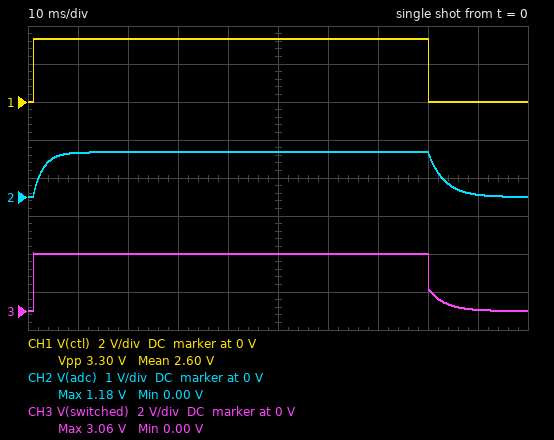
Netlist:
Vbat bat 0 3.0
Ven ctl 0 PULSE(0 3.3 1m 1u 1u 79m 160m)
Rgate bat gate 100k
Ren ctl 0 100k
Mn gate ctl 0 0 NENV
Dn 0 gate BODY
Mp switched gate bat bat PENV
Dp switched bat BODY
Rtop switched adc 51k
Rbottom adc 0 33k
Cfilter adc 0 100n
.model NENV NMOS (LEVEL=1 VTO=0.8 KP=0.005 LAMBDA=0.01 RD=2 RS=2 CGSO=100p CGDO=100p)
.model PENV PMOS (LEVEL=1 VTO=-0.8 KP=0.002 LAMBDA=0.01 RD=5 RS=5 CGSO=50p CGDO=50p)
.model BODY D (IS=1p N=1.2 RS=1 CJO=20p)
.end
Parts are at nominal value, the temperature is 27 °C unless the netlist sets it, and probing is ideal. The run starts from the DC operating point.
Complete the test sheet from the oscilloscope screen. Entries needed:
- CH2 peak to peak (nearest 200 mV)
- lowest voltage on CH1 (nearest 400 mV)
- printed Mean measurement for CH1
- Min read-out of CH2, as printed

1.2 V
0 V
2.60 V
0.00 V
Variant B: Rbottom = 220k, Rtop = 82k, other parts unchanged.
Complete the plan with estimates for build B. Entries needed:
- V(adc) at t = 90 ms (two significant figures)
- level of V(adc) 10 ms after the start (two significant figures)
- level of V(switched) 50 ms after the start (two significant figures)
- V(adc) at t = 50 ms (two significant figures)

1.4 V
1.7 V
3.0 V
2.2 V
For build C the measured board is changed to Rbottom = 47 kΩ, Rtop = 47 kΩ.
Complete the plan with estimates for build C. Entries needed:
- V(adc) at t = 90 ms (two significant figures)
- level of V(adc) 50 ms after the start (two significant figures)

180 mV
1.5 V
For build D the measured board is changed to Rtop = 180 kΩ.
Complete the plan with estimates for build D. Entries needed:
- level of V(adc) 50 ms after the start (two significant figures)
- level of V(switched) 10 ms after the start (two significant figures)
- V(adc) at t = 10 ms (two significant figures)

460 mV
3.0 V
450 mV
